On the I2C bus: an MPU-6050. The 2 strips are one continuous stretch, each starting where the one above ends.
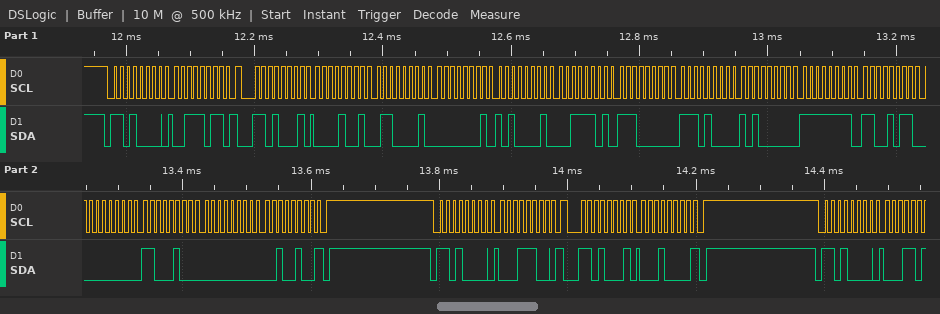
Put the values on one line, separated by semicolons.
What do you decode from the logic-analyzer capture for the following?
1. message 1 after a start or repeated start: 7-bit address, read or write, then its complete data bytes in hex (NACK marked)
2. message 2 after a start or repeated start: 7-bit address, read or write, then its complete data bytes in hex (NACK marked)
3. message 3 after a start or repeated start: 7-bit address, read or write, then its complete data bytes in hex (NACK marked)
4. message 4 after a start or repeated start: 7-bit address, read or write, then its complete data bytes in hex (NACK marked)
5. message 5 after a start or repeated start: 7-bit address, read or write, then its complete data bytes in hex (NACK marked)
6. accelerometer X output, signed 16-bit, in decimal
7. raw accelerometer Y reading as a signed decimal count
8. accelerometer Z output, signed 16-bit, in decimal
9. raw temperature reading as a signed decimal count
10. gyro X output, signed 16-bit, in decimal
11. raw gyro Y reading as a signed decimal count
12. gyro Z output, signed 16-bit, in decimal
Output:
0x68 write: 3B; 0x68 read: 09 61 01 A1 3D E0 E8 A0 FF CB 00 C4 00 24 NACK; 0x68 write: 1C; 0x68 read: 10 NACK; 0x68 write; 2401; 417; 15840; -5984; -53; 196; 36
